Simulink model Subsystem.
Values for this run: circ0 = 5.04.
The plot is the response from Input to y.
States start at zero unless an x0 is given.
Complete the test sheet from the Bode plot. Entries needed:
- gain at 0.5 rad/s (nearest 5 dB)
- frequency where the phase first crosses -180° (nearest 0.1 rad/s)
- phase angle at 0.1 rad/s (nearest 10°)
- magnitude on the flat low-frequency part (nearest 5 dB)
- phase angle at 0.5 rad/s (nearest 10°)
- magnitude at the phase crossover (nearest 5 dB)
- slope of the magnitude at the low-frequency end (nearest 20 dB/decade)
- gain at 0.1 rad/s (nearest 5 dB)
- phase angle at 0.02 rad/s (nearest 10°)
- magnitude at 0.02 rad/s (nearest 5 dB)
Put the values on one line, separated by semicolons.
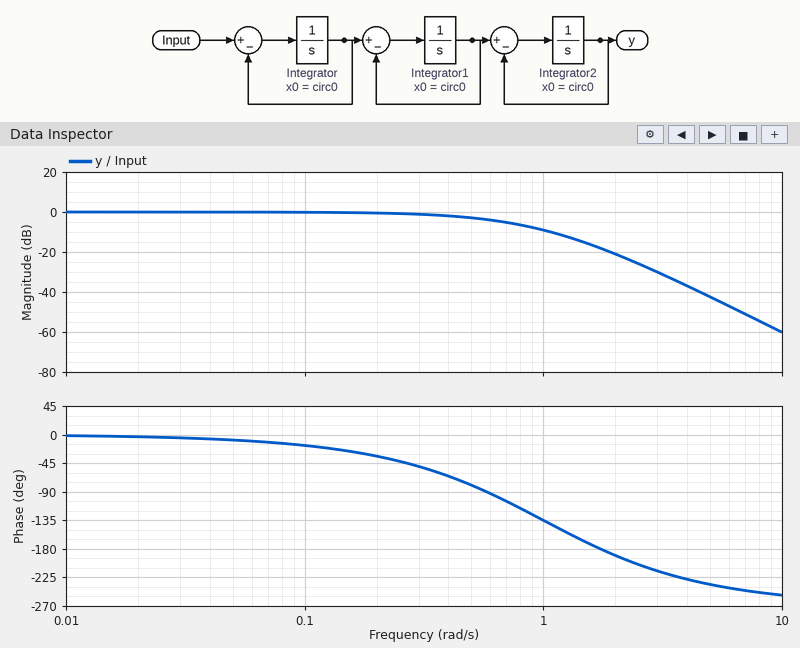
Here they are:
-5 dB; 1.7 rad/s; -20°; 0 dB; -80°; -20 dB; 0 dB/decade; 0 dB; 0°; 0 dB
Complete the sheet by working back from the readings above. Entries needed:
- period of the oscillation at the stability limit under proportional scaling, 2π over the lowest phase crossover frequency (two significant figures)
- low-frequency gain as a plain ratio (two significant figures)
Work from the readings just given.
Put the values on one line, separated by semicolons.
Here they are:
3.7 s; 1.0
